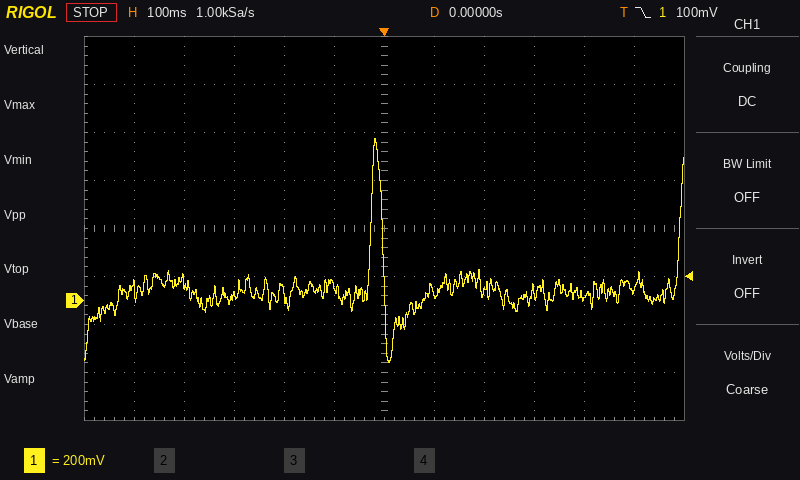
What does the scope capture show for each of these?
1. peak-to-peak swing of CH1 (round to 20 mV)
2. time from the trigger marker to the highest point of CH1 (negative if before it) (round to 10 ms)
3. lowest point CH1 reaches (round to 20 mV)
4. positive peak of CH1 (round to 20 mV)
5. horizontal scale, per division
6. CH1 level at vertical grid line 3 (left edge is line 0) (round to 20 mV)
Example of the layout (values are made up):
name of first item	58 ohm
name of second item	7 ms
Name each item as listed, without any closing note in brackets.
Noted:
peak-to-peak swing of CH1	940 mV
time from the trigger marker to the highest point of CH1 (negative if before it)	-20 ms
lowest point CH1 reaches	-260 mV
positive peak of CH1	680 mV
horizontal scale, per division	100 ms
CH1 level at vertical grid line 3 (left edge is line 0)	20 mV
